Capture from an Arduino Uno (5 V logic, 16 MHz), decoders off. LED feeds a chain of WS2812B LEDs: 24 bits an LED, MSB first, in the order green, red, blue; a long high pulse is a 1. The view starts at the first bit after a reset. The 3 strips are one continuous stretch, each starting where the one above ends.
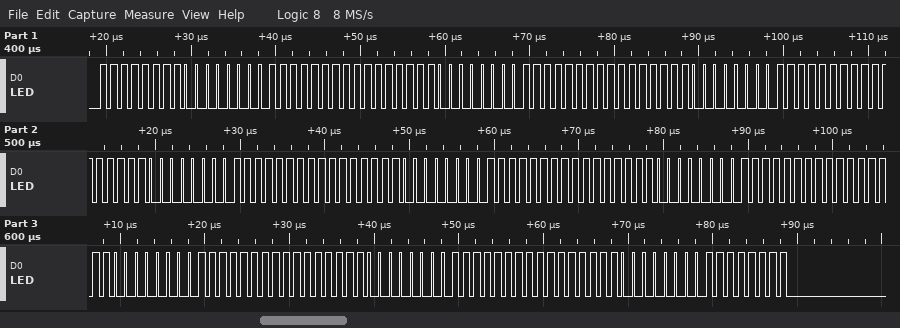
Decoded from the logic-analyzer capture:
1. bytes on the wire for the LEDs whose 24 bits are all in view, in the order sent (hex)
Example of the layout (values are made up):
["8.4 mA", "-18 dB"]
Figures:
["FF 00 FF FF 00 FF FF 00 FF FF 00 FF FF 00 FF FF 00 FF FF 00 FF FF 00 FF FF 00 FF"]
